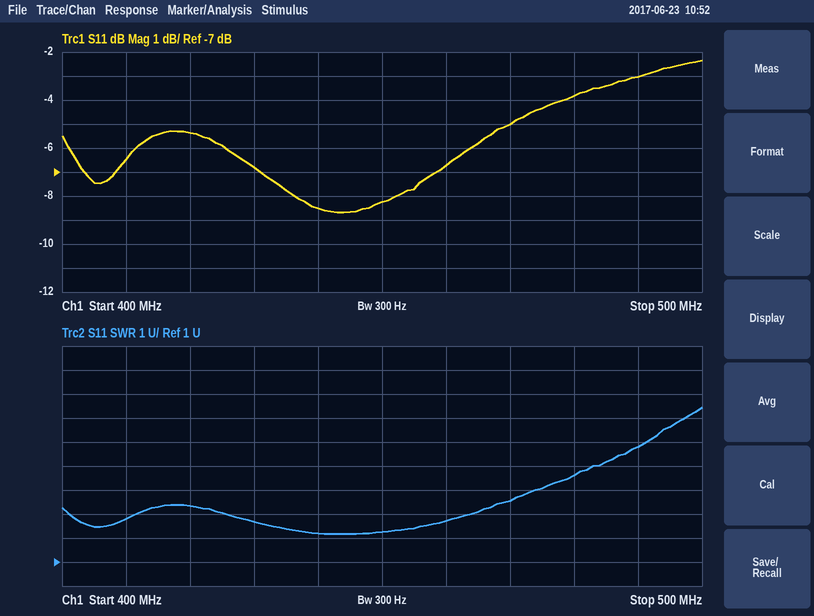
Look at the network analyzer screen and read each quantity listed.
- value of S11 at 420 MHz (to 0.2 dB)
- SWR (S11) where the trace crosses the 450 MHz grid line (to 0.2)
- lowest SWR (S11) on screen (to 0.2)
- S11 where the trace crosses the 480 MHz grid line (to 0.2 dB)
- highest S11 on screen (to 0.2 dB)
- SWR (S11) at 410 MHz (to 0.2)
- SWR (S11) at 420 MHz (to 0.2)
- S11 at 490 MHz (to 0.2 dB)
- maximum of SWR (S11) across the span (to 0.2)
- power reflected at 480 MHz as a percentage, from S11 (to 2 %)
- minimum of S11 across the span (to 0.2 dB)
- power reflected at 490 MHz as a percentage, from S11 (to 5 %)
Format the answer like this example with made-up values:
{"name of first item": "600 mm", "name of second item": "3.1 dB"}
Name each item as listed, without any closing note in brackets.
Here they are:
{"value of S11 at 420 MHz": "-5.4 dB", "SWR (S11) where the trace crosses the 450 MHz grid line": "2.2", "lowest SWR (S11) on screen": "2.2", "S11 where the trace crosses the 480 MHz grid line": "-3.8 dB", "highest S11 on screen": "-2.4 dB", "SWR (S11) at 410 MHz": "2.8", "SWR (S11) at 420 MHz": "3.4", "S11 at 490 MHz": "-3.0 dB", "maximum of SWR (S11) across the span": "7.4", "power reflected at 480 MHz as a percentage, from S11": "42 %", "minimum of S11 across the span": "-8.6 dB", "power reflected at 490 MHz as a percentage, from S11": "50 %"}
